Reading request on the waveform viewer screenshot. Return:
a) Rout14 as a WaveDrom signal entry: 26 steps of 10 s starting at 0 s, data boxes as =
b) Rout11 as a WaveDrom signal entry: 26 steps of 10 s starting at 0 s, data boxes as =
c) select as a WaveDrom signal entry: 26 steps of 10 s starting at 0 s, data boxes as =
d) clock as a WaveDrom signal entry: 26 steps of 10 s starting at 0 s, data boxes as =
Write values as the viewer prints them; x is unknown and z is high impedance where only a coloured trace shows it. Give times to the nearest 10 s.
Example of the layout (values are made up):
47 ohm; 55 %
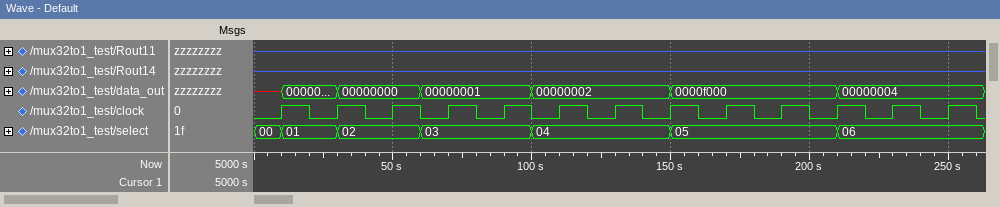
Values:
{name: 'Rout14', wave: 'z.........................'}; {name: 'Rout11', wave: 'z.........................'}; {name: 'select', wave: '==.=..=...=....=.....=....', data: '00 01 02 03 04 05 06'}; {name: 'clock', wave: '01010101010101010101010101'}
